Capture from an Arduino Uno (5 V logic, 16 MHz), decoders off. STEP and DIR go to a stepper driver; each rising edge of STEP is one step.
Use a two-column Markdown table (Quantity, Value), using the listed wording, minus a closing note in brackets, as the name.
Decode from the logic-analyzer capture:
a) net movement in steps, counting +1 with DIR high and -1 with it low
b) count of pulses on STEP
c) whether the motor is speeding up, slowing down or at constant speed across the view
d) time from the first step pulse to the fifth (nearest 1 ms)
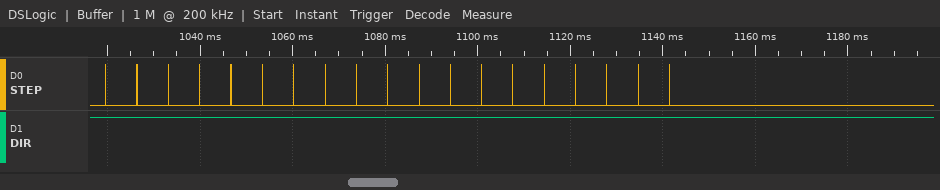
| Quantity | Value |
|---|---|
| net movement in steps, counting +1 with DIR high and -1 with it low | +19 |
| count of pulses on STEP | 19 |
| whether the motor is speeding up, slowing down or at constant speed across the view | constant speed |
| time from the first step pulse to the fifth | 27 ms |
